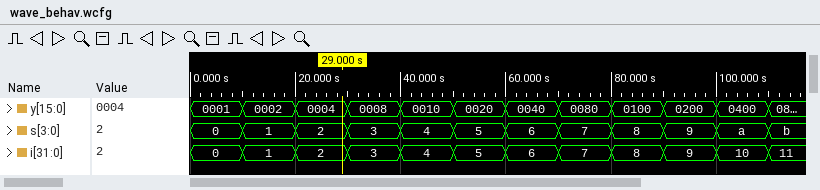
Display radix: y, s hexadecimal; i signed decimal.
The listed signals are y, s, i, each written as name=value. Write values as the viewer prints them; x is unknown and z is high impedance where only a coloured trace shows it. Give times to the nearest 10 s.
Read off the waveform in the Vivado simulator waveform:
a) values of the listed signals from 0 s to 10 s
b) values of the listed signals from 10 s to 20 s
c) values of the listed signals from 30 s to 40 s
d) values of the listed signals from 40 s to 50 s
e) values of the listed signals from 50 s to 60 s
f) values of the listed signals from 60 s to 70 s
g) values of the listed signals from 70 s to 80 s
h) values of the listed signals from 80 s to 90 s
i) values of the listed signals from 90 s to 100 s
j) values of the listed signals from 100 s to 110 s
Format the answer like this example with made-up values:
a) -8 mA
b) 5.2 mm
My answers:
a) y=0001, s=0, i=0
b) y=0002, s=1, i=1
c) y=0008, s=3, i=3
d) y=0010, s=4, i=4
e) y=0020, s=5, i=5
f) y=0040, s=6, i=6
g) y=0080, s=7, i=7
h) y=0100, s=8, i=8
i) y=0200, s=9, i=9
j) y=0400, s=a, i=10
